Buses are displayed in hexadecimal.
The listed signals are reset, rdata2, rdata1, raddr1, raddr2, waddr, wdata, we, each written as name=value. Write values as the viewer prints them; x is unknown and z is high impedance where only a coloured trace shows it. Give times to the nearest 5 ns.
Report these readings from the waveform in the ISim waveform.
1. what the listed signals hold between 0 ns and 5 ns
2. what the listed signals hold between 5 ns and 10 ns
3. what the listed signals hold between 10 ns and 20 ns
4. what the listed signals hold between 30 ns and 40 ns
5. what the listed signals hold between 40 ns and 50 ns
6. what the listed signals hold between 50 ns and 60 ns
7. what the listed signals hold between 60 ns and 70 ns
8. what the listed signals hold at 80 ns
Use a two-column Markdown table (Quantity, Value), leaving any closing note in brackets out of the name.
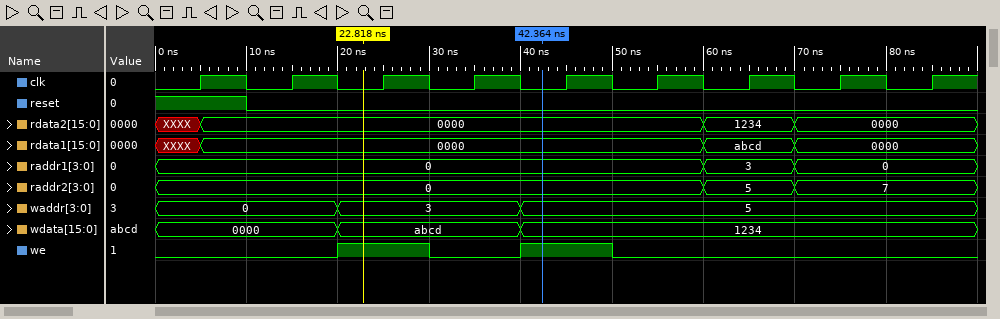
| Quantity | Value |
|---|---|
| what the listed signals hold between 0 ns and 5 ns | reset=1, rdata2=XXXX, rdata1=XXXX, raddr1=0, raddr2=0, waddr=0, wdata=0000, we=0 |
| what the listed signals hold between 5 ns and 10 ns | reset=1, rdata2=0000, rdata1=0000, raddr1=0, raddr2=0, waddr=0, wdata=0000, we=0 |
| what the listed signals hold between 10 ns and 20 ns | reset=0, rdata2=0000, rdata1=0000, raddr1=0, raddr2=0, waddr=0, wdata=0000, we=0 |
| what the listed signals hold between 30 ns and 40 ns | reset=0, rdata2=0000, rdata1=0000, raddr1=0, raddr2=0, waddr=3, wdata=abcd, we=0 |
| what the listed signals hold between 40 ns and 50 ns | reset=0, rdata2=0000, rdata1=0000, raddr1=0, raddr2=0, waddr=5, wdata=1234, we=1 |
| what the listed signals hold between 50 ns and 60 ns | reset=0, rdata2=0000, rdata1=0000, raddr1=0, raddr2=0, waddr=5, wdata=1234, we=0 |
| what the listed signals hold between 60 ns and 70 ns | reset=0, rdata2=1234, rdata1=abcd, raddr1=3, raddr2=5, waddr=5, wdata=1234, we=0 |
| what the listed signals hold at 80 ns | reset=0, rdata2=0000, rdata1=0000, raddr1=0, raddr2=7, waddr=5, wdata=1234, we=0 |
